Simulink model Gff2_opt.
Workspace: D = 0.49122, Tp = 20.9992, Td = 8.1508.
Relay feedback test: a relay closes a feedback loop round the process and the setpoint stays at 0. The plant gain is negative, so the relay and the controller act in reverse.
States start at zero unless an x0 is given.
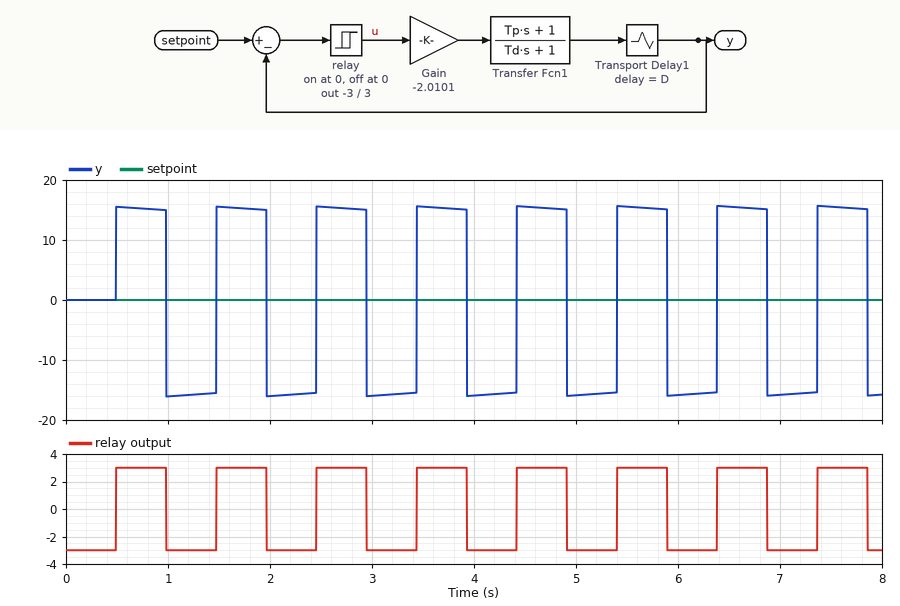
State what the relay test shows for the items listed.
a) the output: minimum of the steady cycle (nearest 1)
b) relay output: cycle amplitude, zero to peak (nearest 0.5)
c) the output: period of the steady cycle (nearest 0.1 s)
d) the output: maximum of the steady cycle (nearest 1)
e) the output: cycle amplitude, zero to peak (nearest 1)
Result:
-16
3.0
1.0 s
16
16
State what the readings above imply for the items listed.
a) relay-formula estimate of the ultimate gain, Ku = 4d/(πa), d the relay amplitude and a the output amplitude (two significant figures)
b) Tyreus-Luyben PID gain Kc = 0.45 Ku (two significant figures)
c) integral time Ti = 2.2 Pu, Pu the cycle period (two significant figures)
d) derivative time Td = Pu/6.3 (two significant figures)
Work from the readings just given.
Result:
0.24
0.11
2.2 s
0.16 s
